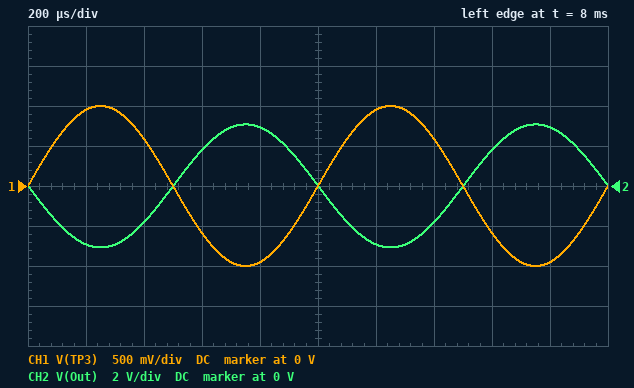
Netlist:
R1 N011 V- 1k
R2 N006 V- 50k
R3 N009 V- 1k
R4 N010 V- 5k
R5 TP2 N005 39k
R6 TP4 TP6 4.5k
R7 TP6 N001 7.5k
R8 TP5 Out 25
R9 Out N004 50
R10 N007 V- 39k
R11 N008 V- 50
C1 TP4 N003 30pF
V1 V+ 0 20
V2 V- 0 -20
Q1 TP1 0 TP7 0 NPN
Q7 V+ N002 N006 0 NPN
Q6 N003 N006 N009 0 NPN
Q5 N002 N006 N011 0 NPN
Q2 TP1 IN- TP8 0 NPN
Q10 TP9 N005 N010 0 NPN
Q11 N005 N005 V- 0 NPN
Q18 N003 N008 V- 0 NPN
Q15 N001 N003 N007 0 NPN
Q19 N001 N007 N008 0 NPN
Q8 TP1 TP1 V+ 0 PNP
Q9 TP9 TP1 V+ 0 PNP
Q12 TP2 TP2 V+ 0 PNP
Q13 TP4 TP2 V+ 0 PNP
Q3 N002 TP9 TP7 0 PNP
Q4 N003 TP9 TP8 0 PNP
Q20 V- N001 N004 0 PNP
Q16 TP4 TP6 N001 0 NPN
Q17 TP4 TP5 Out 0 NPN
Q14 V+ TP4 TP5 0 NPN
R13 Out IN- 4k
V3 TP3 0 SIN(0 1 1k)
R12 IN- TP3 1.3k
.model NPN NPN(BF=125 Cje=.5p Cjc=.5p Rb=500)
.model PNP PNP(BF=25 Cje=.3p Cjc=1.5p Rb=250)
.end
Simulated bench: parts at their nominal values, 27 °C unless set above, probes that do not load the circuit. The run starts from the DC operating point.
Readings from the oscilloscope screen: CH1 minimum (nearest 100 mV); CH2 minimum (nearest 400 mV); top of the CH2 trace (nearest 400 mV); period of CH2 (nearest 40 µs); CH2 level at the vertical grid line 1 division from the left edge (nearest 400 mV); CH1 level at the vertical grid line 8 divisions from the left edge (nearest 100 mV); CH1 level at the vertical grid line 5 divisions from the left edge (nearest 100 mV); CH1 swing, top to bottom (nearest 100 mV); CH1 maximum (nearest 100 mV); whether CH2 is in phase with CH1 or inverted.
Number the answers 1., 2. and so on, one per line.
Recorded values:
1. -1.0 V
2. -3.2 V
3. 3.2 V
4. 1.00 ms
5. -2.8 V
6. -600 mV
7. 0 V
8. 2.0 V
9. 1.0 V
10. inverted
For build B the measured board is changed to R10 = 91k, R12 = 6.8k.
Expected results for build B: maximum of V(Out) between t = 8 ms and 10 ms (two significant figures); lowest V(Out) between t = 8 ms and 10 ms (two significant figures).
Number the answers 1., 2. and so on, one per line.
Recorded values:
1. 590 mV
2. -590 mV
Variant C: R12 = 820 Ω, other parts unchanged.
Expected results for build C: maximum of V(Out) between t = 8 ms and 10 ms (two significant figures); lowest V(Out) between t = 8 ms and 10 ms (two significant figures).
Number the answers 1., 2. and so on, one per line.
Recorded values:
1. 4.9 V
2. -4.9 V
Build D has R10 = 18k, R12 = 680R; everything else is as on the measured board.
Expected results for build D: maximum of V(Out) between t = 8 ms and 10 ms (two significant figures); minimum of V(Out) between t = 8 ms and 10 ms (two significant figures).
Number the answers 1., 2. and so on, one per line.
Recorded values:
1. 5.9 V
2. -5.9 V
